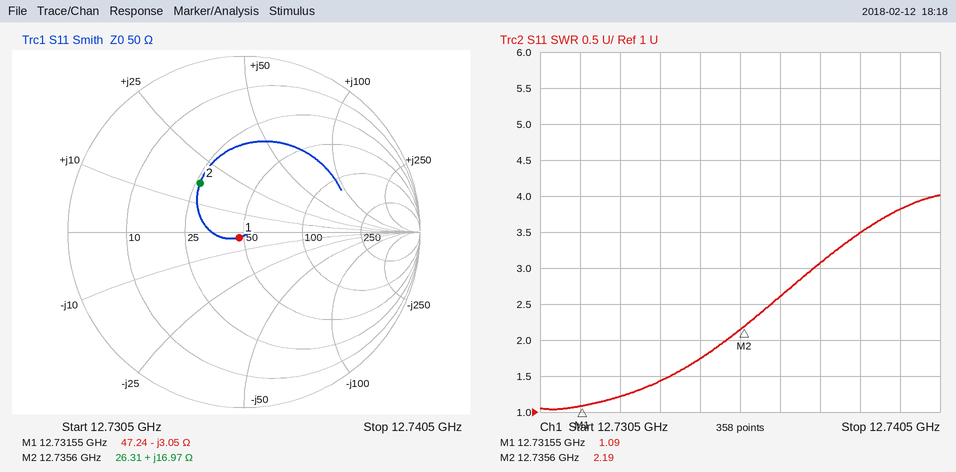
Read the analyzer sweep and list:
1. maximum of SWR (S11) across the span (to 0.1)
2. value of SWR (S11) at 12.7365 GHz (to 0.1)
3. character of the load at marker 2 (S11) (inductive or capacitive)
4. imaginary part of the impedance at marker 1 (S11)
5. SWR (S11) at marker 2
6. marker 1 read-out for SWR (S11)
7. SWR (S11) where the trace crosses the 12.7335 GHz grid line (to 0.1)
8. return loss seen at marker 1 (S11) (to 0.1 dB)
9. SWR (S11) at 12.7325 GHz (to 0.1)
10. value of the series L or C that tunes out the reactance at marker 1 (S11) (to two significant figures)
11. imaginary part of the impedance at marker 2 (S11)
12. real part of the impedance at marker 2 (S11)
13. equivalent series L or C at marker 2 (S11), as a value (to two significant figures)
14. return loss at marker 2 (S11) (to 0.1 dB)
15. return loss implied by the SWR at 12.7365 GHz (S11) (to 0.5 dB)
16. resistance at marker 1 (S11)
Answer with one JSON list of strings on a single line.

["4.0", "2.6", "inductive", "-3.05 Ω", "2.19", "1.09", "1.4", "27.5 dB", "1.2", "38 pH", "+16.97 Ω", "26.31 Ω", "210 pH", "8.6 dB", "7.0 dB", "47.24 Ω"]
